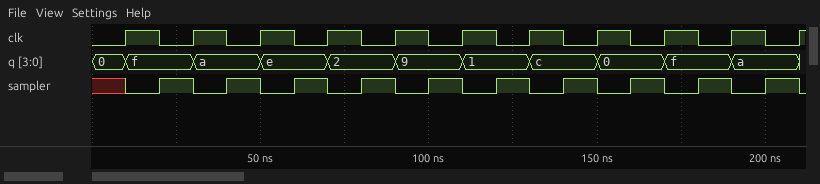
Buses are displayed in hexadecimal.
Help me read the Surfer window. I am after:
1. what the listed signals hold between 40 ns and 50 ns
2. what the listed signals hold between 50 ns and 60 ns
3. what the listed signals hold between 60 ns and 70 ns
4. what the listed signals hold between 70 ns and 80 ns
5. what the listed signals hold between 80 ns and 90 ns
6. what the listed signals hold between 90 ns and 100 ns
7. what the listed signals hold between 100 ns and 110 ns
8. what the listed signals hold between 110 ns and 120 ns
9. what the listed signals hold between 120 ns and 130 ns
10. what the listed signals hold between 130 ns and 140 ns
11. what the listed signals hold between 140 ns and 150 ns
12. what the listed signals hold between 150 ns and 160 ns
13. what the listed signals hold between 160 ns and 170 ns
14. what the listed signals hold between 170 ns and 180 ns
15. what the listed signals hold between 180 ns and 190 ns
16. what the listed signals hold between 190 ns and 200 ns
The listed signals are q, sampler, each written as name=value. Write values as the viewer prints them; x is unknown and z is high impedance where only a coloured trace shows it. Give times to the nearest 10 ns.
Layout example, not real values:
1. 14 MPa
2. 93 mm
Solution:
1. q=a, sampler=1
2. q=e, sampler=0
3. q=e, sampler=1
4. q=2, sampler=0
5. q=2, sampler=1
6. q=9, sampler=0
7. q=9, sampler=1
8. q=1, sampler=0
9. q=1, sampler=1
10. q=c, sampler=0
11. q=c, sampler=1
12. q=0, sampler=0
13. q=0, sampler=1
14. q=f, sampler=0
15. q=f, sampler=1
16. q=a, sampler=0
